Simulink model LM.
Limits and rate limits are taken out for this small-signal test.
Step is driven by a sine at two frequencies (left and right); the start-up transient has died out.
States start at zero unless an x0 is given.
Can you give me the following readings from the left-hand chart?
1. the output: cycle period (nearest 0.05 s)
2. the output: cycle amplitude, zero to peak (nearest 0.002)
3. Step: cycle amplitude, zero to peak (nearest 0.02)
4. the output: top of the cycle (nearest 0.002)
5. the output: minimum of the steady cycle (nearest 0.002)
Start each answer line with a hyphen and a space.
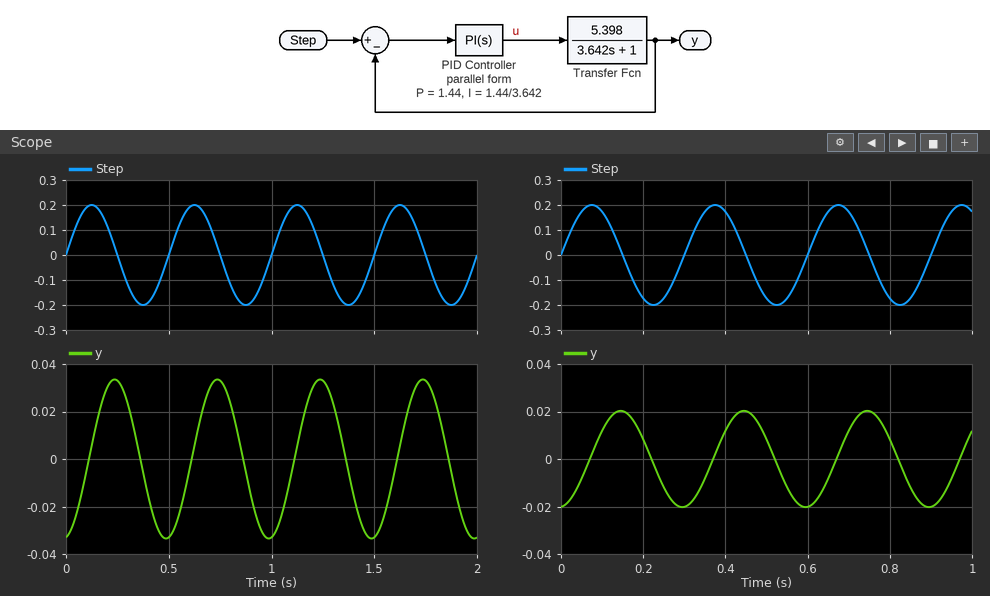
- 0.50 s
- 0.034
- 0.20
- 0.034
- -0.034
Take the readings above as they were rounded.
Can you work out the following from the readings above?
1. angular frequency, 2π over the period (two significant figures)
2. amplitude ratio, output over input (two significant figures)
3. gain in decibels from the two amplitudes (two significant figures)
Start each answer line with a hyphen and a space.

- 13 rad/s
- 0.17
- -15 dB
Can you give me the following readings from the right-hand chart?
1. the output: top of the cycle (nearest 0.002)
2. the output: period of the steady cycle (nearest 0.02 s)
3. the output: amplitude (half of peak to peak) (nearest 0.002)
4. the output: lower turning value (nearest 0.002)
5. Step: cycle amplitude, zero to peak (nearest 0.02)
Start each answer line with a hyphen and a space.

- 0.020
- 0.30 s
- 0.020
- -0.020
- 0.20
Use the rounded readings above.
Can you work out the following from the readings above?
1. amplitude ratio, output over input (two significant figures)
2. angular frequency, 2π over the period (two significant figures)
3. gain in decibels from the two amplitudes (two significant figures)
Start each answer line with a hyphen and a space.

- 0.10
- 21 rad/s
- -20 dB
